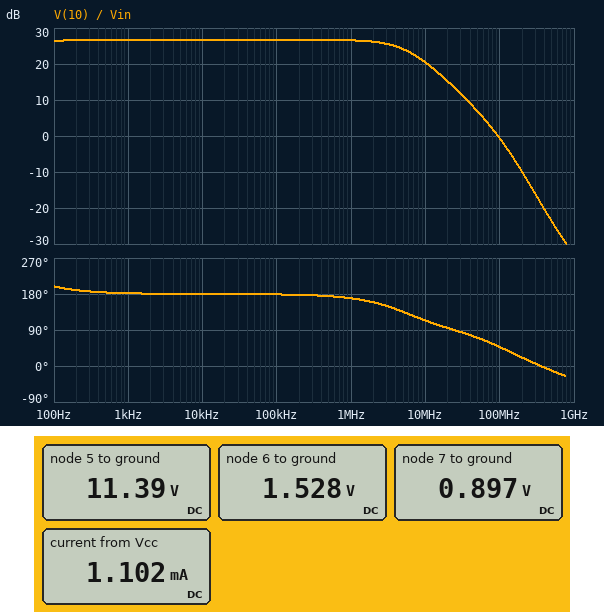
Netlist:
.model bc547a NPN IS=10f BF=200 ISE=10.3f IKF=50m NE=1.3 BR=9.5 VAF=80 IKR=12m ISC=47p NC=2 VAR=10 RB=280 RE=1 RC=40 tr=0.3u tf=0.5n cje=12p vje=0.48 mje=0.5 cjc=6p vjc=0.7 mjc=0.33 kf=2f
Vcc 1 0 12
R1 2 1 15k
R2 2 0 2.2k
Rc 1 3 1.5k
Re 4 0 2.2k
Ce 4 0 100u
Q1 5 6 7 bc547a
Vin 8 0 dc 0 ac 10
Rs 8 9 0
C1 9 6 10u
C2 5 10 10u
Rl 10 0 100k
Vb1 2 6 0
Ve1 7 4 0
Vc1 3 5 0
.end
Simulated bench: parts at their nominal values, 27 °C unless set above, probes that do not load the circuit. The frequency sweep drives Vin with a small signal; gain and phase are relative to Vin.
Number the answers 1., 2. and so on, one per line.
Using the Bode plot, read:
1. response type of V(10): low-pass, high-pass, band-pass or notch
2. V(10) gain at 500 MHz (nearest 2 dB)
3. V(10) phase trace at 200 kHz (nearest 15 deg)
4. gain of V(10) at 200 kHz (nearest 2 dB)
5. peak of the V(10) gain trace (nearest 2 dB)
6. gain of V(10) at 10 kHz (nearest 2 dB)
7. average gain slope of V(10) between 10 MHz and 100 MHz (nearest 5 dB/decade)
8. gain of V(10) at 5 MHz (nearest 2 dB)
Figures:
1. low-pass
2. -24 dB
3. 180 deg
4. 26 dB
5. 26 dB
6. 26 dB
7. -20 dB/decade
8. 24 dB
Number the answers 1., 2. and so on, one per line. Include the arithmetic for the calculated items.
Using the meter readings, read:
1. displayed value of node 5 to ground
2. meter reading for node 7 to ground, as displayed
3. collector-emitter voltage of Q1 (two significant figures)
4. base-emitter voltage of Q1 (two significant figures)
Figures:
1. 11.39 V
2. 0.897 V
3. 11.39 V - 897 mV = 10 V
4. 1.528 V - 897 mV = 630 mV
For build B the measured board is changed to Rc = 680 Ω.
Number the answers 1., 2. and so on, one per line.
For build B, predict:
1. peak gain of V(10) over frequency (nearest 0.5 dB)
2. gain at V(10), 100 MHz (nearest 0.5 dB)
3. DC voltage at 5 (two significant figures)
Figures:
1. 20.0 dB
2. -3.0 dB
3. 12 V
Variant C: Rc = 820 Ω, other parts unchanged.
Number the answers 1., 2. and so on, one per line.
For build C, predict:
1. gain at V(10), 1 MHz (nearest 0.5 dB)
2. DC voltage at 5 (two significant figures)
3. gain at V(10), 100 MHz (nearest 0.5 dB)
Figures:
1. 21.5 dB
2. 12 V
3. -2.0 dB
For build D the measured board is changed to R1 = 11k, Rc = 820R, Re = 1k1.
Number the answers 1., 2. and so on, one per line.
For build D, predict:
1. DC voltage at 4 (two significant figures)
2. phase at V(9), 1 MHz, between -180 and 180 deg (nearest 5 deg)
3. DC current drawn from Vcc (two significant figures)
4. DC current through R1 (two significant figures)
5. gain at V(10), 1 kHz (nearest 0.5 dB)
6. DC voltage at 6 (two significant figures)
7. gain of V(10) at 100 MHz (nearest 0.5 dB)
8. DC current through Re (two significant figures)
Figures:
1. 1.3 V
2. 0 deg
3. 2.1 mA
4. 910 µA
5. 30.0 dB
6. 2.0 V
7. 1.5 dB
8. 1.2 mA
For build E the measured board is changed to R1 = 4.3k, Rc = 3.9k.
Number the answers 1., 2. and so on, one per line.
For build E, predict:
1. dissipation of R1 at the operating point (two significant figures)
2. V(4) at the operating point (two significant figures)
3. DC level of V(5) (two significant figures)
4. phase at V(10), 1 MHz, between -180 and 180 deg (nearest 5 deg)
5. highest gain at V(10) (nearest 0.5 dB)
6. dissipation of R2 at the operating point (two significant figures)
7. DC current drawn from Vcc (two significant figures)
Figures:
1. 15 mW
2. 3.4 V
3. 6.1 V
4. 125 deg
5. 44.5 dB
6. 7.4 mW
7. 3.4 mA
